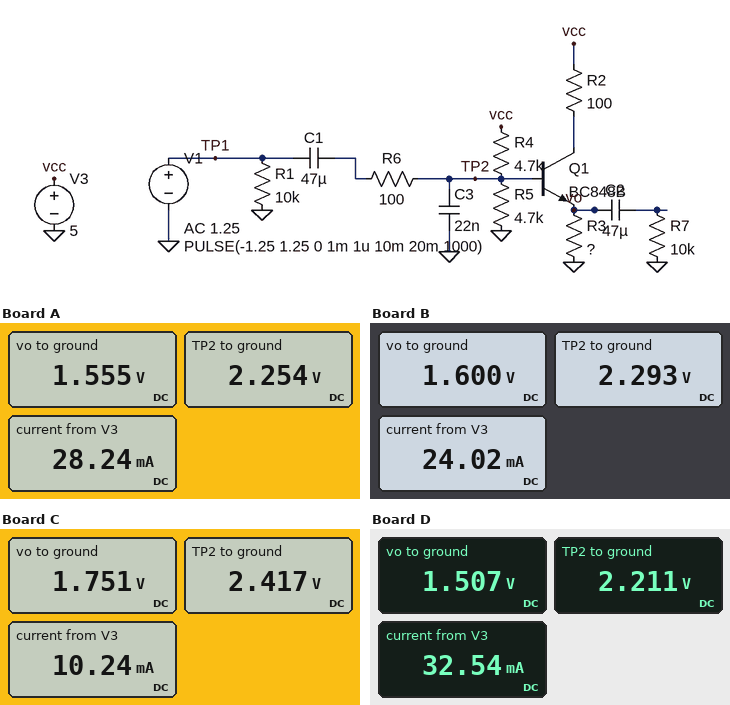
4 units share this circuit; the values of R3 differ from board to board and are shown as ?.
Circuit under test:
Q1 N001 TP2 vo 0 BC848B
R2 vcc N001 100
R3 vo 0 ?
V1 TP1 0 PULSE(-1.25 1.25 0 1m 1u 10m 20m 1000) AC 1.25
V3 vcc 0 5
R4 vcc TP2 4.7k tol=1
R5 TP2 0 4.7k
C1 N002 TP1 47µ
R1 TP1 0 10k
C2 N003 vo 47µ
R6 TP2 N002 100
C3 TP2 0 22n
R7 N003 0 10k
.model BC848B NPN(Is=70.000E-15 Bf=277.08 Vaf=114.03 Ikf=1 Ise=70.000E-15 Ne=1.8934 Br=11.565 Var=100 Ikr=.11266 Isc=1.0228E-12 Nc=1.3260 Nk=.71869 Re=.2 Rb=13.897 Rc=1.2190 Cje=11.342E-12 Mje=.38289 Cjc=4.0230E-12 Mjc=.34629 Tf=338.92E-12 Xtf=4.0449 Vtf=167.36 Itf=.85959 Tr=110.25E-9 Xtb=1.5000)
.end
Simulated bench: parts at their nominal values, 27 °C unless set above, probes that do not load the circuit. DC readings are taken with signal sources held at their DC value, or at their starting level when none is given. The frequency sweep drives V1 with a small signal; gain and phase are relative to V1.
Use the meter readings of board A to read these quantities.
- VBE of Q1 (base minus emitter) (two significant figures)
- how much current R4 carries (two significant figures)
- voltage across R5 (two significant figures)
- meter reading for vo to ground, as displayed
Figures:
700 mV
580 µA
2.3 V
1.555 V
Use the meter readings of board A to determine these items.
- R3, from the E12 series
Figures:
56 Ω
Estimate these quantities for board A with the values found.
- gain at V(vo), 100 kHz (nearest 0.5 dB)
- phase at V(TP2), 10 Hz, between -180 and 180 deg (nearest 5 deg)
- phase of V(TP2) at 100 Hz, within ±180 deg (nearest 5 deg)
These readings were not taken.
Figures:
-5.0 dB
10 deg
0 deg
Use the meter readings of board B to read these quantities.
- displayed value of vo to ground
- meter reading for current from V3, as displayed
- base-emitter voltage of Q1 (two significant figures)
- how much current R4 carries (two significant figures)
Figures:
1.600 V
24.02 mA
690 mV
580 µA
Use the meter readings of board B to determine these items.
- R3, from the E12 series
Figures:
68 Ω
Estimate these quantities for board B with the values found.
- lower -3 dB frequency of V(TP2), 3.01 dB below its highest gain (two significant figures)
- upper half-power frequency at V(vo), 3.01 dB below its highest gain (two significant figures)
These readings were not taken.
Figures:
1.6 Hz
76 kHz
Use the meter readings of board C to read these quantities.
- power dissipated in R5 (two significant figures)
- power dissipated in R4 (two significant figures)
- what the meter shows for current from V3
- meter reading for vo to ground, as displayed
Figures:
1.2 mW
1.4 mW
10.24 mA
1.751 V
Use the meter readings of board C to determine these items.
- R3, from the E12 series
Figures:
180 Ω
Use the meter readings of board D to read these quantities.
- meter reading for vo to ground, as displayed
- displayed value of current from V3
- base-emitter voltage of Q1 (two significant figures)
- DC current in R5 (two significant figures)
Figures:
1.507 V
32.54 mA
700 mV
470 µA
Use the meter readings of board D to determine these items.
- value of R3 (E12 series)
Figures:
47 Ω
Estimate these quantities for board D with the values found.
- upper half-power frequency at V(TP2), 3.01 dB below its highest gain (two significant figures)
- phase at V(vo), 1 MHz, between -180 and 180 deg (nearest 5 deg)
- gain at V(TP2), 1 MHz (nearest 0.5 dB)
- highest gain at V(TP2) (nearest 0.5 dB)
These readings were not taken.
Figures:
76 kHz
-85 deg
-23.0 dB
-0.5 dB
